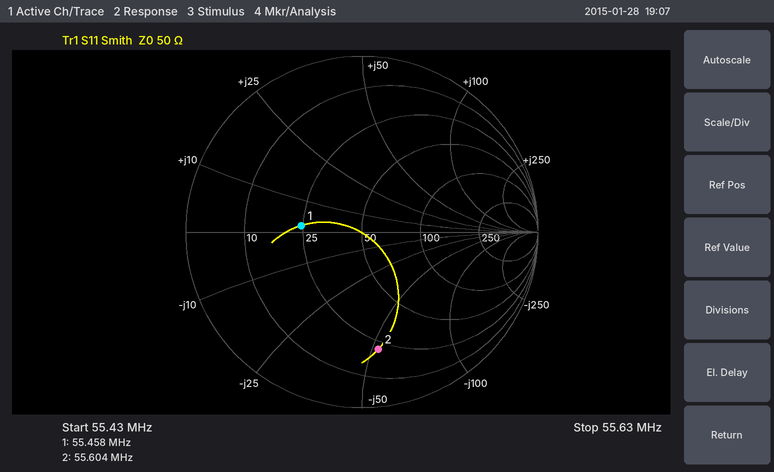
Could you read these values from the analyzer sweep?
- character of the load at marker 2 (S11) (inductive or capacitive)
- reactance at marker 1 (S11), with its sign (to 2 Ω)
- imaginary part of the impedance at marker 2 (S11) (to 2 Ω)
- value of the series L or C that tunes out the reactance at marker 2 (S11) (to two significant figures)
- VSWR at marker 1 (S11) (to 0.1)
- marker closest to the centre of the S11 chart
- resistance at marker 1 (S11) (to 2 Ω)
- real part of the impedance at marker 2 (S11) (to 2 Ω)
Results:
capacitive
+2 Ω
-52 Ω
150 nH
2.1
marker 1
24 Ω
22 Ω
